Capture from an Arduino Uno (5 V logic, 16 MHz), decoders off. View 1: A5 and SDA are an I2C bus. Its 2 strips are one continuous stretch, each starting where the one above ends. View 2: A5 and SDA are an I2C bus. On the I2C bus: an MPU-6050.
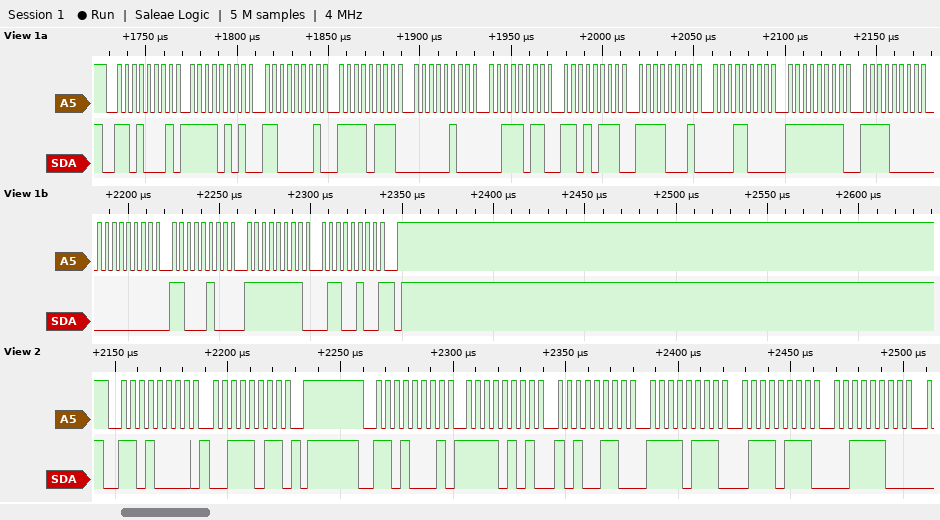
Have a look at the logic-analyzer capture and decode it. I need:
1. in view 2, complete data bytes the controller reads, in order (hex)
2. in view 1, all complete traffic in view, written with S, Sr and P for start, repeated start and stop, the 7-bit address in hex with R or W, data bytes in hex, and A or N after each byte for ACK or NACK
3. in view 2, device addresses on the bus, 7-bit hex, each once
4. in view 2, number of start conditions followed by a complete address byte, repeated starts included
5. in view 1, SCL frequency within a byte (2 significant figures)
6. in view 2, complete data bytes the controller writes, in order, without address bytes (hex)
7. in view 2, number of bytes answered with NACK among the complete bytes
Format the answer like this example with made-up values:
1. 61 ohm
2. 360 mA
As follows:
1. F5 A6 F7 77 3C
2. S 68R A F5 A C1 A F7 A 04 A 3B A D7 A F1 A 18 A FF A F0 A 00 A C4 A FF A 64 N P
3. 0x68
4. 2
5. 250 kHz
6. 3B
7. 0
